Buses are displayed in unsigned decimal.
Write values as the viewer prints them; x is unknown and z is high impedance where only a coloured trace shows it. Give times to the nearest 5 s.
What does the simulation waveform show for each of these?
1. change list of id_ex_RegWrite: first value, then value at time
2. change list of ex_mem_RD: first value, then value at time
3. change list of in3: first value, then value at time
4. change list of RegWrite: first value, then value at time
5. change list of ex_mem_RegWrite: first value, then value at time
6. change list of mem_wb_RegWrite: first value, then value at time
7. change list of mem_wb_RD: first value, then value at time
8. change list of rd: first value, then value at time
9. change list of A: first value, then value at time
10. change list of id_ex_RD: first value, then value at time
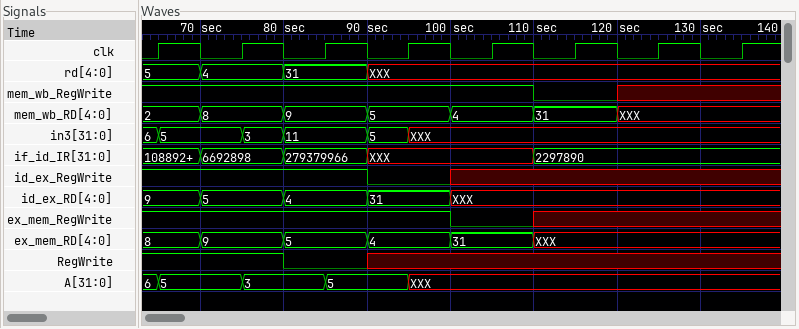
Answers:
1, 0 at 90 s, x at 100 s
8, 9 at 70 s, 5 at 80 s, 4 at 90 s, 31 at 100 s, XXX at 110 s
6, 5 at 65 s, 3 at 75 s, 11 at 80 s, 5 at 90 s, XXX at 95 s
1, 0 at 80 s, x at 90 s
1, 0 at 100 s, x at 110 s
1, 0 at 110 s, x at 120 s
2, 8 at 70 s, 9 at 80 s, 5 at 90 s, 4 at 100 s, 31 at 110 s, XXX at 120 s
5, 4 at 70 s, 31 at 80 s, XXX at 90 s
6, 5 at 65 s, 3 at 75 s, 5 at 85 s, XXX at 95 s
9, 5 at 70 s, 4 at 80 s, 31 at 90 s, XXX at 100 s
